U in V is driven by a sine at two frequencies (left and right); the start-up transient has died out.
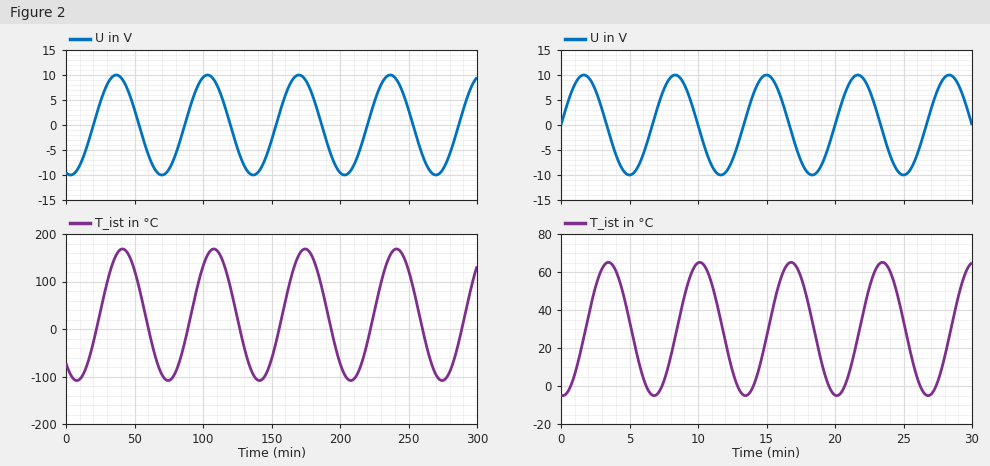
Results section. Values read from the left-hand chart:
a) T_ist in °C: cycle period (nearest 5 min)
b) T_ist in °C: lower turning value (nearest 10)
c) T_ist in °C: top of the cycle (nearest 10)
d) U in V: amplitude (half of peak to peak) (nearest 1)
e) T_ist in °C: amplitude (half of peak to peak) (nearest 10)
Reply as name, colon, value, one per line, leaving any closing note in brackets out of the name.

T_ist in °C: cycle period: 65 min
T_ist in °C: lower turning value: -110
T_ist in °C: top of the cycle: 170
U in V: amplitude (half of peak to peak): 10
T_ist in °C: amplitude (half of peak to peak): 140
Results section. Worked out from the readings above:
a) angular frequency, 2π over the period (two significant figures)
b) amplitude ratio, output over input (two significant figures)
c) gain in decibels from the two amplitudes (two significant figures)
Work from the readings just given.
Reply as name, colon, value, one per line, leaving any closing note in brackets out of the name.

angular frequency, 2π over the period: 0.097 rad/min
amplitude ratio, output over input: 14
gain in decibels from the two amplitudes: 23 dB
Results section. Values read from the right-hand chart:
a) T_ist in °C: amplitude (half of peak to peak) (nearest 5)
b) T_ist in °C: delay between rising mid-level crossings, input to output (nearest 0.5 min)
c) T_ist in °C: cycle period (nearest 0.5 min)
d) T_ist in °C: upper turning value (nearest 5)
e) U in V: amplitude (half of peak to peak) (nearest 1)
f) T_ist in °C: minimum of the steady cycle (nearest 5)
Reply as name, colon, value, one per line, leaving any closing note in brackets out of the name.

T_ist in °C: amplitude (half of peak to peak): 35
T_ist in °C: delay between rising mid-level crossings, input to output: 2.0 min
T_ist in °C: cycle period: 6.5 min
T_ist in °C: upper turning value: 65
U in V: amplitude (half of peak to peak): 10
T_ist in °C: minimum of the steady cycle: -5
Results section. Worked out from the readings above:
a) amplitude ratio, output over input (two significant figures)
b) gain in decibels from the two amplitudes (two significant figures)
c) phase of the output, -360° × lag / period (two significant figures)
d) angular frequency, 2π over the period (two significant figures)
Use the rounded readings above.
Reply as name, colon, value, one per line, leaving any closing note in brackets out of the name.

amplitude ratio, output over input: 3.5
gain in decibels from the two amplitudes: 11 dB
phase of the output, -360° × lag / period: -110°
angular frequency, 2π over the period: 0.97 rad/min
